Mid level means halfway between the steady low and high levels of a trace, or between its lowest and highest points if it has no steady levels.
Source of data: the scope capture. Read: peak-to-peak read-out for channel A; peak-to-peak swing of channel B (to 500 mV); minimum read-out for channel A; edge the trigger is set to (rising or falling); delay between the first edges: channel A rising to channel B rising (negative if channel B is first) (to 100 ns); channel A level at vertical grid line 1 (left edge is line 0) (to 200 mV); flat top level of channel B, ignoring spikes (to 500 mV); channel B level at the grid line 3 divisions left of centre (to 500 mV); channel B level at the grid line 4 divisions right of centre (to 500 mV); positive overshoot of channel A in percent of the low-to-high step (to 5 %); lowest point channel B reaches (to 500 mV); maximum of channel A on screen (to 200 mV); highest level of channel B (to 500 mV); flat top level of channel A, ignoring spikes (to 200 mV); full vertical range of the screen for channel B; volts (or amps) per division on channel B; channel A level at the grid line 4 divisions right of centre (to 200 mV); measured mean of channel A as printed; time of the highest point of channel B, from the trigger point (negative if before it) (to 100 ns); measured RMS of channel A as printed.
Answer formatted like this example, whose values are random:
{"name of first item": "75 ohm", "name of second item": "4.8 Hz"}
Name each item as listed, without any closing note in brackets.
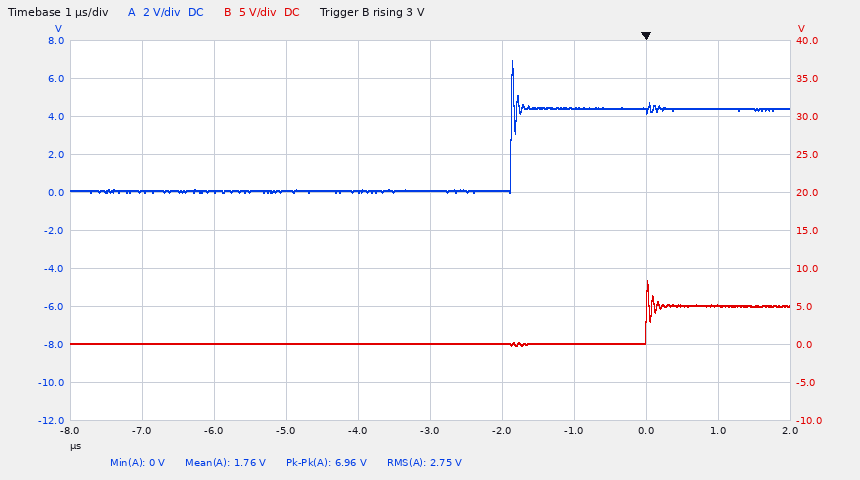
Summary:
{"peak-to-peak read-out for channel A": "6.96 V", "peak-to-peak swing of channel B": "8.5 V", "minimum read-out for channel A": "0 V", "edge the trigger is set to": "rising", "delay between the first edges: channel A rising to channel B rising (negative if channel B is first)": "+1.9 µs", "channel A level at vertical grid line 1 (left edge is line 0)": "0.0 V", "flat top level of channel B, ignoring spikes": "5.0 V", "channel B level at the grid line 3 divisions left of centre": "0.0 V", "channel B level at the grid line 4 divisions right of centre": "5.0 V", "positive overshoot of channel A in percent of the low-to-high step": "60 %", "lowest point channel B reaches": "0.0 V", "maximum of channel A on screen": "7.0 V", "highest level of channel B": "8.5 V", "flat top level of channel A, ignoring spikes": "4.4 V", "full vertical range of the screen for channel B": "50 V", "volts (or amps) per division on channel B": "5 V", "channel A level at the grid line 4 divisions right of centre": "4.4 V", "measured mean of channel A as printed": "1.76 V", "time of the highest point of channel B, from the trigger point (negative if before it)": "0.0 µs", "measured RMS of channel A as printed": "2.75 V"}
